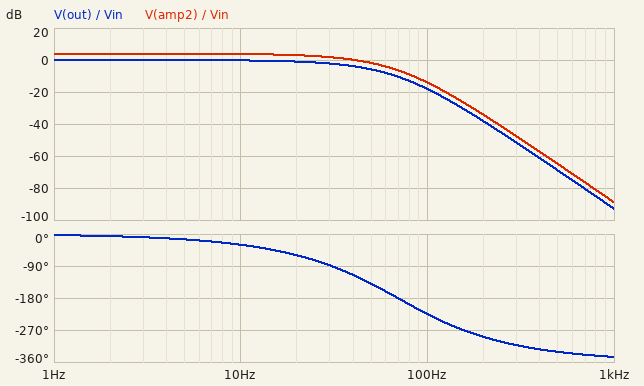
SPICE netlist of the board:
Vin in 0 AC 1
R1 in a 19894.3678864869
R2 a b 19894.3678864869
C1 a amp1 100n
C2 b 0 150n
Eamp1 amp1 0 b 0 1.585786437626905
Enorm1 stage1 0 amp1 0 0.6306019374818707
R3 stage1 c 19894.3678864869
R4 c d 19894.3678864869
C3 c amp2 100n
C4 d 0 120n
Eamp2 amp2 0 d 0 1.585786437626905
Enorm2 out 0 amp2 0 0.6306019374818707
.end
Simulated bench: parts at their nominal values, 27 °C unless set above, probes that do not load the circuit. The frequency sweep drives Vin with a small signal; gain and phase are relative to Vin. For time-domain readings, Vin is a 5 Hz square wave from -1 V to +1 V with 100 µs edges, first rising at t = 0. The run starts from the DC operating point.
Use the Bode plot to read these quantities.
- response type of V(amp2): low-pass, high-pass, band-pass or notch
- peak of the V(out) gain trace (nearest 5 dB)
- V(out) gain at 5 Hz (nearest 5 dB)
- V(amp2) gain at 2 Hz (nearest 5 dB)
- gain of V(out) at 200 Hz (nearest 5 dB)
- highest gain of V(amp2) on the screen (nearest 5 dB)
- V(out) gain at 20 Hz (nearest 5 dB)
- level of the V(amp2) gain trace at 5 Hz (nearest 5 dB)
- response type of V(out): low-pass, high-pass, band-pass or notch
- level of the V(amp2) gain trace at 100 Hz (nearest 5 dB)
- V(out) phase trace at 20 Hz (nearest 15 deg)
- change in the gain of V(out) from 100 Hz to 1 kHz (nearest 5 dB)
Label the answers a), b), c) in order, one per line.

a) low-pass
b) 0 dB
c) 0 dB
d) 5 dB
e) -40 dB
f) 5 dB
g) 0 dB
h) 5 dB
i) low-pass
j) -15 dB
k) -60 deg
l) -75 dB
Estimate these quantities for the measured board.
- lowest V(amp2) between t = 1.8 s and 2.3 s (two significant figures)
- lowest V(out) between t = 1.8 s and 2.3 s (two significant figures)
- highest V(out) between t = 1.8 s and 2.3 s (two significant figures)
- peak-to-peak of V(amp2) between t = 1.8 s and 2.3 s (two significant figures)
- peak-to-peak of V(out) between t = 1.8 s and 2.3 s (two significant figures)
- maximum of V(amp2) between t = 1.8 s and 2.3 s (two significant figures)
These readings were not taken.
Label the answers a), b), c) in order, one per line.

a) -1.6 V
b) -1.0 V
c) 1.0 V
d) 3.2 V
e) 2.0 V
f) 1.6 V
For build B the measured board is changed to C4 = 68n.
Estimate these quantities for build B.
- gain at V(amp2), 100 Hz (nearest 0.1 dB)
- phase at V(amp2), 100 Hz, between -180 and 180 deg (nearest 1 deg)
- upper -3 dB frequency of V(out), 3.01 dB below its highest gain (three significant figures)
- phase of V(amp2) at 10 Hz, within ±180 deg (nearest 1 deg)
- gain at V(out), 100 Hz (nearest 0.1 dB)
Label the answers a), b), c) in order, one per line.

a) -6.1 dB
b) 152 deg
c) 52.5 Hz
d) -23 deg
e) -10.1 dB
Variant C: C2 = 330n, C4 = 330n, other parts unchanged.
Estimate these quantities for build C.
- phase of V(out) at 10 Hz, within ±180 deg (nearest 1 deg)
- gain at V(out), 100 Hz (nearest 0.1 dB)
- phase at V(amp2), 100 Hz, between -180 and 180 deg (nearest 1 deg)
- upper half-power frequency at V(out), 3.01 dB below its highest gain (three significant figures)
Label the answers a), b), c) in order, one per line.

a) -77 deg
b) -37.4 dB
c) 122 deg
d) 9.44 Hz
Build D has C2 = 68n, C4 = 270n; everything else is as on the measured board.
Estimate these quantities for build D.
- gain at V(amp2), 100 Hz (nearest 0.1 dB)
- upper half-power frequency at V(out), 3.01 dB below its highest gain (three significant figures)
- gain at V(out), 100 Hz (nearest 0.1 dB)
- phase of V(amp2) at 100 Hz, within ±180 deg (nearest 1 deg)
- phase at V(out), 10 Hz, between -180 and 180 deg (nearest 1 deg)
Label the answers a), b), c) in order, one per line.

a) -12.4 dB
b) 19.6 Hz
c) -16.4 dB
d) 148 deg
e) -38 deg
